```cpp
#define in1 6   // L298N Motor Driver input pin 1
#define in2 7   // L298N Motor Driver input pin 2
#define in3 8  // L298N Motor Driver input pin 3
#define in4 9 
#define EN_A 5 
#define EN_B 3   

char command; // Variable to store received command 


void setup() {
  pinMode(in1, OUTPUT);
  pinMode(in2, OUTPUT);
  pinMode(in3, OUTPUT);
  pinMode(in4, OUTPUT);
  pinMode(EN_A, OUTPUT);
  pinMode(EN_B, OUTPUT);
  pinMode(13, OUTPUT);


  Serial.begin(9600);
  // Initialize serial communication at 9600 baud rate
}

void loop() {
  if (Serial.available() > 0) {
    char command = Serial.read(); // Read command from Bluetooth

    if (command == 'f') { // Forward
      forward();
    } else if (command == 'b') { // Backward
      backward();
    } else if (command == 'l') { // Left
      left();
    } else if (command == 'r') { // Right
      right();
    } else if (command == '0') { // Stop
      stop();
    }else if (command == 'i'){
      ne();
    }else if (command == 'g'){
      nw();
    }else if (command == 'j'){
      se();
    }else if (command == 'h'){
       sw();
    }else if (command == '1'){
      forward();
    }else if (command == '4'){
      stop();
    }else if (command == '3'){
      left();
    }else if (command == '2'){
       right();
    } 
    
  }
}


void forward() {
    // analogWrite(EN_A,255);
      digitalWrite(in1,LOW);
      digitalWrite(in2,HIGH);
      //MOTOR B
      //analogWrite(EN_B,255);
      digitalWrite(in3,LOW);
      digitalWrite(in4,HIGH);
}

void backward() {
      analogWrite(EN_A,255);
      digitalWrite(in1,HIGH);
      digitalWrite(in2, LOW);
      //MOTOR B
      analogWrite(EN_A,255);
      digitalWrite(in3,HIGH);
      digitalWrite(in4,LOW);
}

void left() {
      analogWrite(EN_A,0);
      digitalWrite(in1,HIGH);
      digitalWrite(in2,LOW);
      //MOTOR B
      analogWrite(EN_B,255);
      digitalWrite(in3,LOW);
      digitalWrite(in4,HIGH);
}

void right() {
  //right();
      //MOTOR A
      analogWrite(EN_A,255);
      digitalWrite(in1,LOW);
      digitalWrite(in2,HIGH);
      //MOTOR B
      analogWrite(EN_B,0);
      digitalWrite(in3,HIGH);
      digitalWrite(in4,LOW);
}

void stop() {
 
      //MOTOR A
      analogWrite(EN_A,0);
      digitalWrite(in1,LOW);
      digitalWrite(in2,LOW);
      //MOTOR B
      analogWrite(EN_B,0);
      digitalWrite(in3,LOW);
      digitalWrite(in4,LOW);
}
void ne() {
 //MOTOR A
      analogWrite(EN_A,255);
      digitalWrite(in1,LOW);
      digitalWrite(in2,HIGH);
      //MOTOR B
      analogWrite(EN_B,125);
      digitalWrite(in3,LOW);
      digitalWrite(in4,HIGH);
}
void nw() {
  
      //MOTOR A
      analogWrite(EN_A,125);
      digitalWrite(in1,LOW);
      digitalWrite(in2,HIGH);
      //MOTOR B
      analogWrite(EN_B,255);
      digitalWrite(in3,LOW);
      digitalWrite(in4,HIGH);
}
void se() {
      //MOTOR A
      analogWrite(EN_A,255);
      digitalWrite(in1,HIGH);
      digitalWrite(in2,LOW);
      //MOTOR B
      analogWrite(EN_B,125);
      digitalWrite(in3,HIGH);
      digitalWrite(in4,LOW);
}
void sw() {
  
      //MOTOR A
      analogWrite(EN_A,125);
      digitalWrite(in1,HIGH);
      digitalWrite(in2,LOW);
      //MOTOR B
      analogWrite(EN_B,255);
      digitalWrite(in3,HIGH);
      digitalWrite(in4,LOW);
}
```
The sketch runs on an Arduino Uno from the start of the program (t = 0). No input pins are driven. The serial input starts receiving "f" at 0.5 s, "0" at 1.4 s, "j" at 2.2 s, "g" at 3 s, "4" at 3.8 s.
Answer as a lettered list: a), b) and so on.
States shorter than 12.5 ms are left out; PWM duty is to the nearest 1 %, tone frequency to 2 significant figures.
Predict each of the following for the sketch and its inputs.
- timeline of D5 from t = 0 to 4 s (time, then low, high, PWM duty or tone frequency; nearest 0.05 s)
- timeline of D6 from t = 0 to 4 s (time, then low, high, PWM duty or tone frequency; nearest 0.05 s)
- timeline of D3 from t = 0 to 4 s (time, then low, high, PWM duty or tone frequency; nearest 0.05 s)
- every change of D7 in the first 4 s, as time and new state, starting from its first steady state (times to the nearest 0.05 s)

a) 0 s low; 2.2 s high; 3 s PWM 49 %; 3.8 s low
b) 0 s low; 2.2 s high; 3 s low
c) 0 s low; 2.2 s PWM 49 %; 3 s high; 3.8 s low
d) 0 s low; 0.5 s high; 1.4 s low; 3 s high; 3.8 s low
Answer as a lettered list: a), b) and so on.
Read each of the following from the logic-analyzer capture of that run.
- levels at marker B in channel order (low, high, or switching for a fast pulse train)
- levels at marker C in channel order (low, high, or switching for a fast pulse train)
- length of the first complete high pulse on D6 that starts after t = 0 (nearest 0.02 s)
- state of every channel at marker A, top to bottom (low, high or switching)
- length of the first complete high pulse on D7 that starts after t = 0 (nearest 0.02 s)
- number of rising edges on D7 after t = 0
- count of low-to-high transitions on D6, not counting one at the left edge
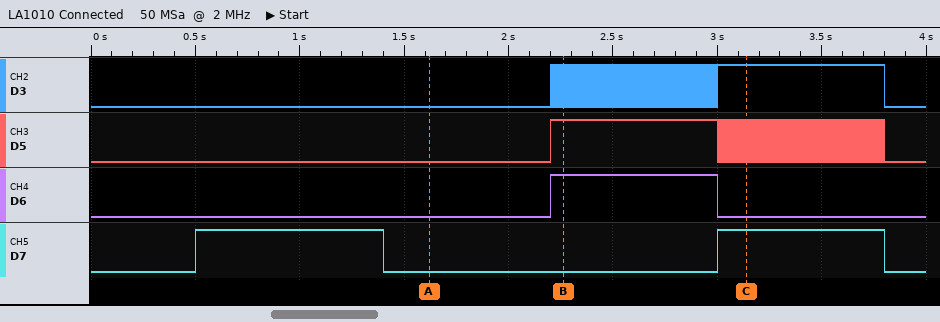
a) D3 switching, D5 high, D6 high, D7 low
b) D3 high, D5 switching, D6 low, D7 high
c) 0.80 s
d) D3 low, D5 low, D6 low, D7 low
e) 0.90 s
f) 2
g) 1
